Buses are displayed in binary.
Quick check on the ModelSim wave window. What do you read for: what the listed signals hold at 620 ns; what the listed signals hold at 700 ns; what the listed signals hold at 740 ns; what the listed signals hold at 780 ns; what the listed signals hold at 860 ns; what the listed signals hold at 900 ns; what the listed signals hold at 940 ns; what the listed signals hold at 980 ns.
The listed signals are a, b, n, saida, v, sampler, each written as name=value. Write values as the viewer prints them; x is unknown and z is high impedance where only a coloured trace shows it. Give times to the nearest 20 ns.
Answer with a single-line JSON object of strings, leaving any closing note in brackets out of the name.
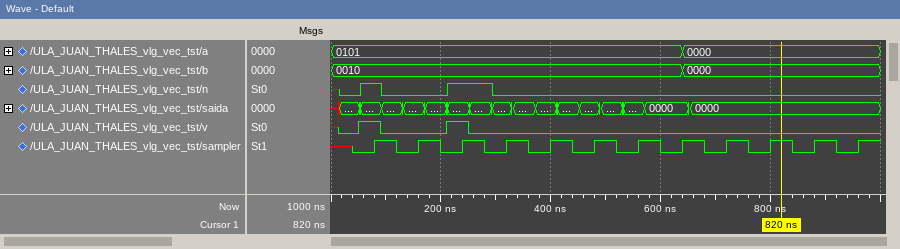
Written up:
{"what the listed signals hold at 620 ns": "a=0101, b=0010, n=0, saida=0000, v=0, sampler=0", "what the listed signals hold at 700 ns": "a=0000, b=0000, n=0, saida=0000, v=0, sampler=0", "what the listed signals hold at 740 ns": "a=0000, b=0000, n=0, saida=0000, v=0, sampler=1", "what the listed signals hold at 780 ns": "a=0000, b=0000, n=0, saida=0000, v=0, sampler=0", "what the listed signals hold at 860 ns": "a=0000, b=0000, n=0, saida=0000, v=0, sampler=0", "what the listed signals hold at 900 ns": "a=0000, b=0000, n=0, saida=0000, v=0, sampler=1", "what the listed signals hold at 940 ns": "a=0000, b=0000, n=0, saida=0000, v=0, sampler=0", "what the listed signals hold at 980 ns": "a=0000, b=0000, n=0, saida=0000, v=0, sampler=1"}
